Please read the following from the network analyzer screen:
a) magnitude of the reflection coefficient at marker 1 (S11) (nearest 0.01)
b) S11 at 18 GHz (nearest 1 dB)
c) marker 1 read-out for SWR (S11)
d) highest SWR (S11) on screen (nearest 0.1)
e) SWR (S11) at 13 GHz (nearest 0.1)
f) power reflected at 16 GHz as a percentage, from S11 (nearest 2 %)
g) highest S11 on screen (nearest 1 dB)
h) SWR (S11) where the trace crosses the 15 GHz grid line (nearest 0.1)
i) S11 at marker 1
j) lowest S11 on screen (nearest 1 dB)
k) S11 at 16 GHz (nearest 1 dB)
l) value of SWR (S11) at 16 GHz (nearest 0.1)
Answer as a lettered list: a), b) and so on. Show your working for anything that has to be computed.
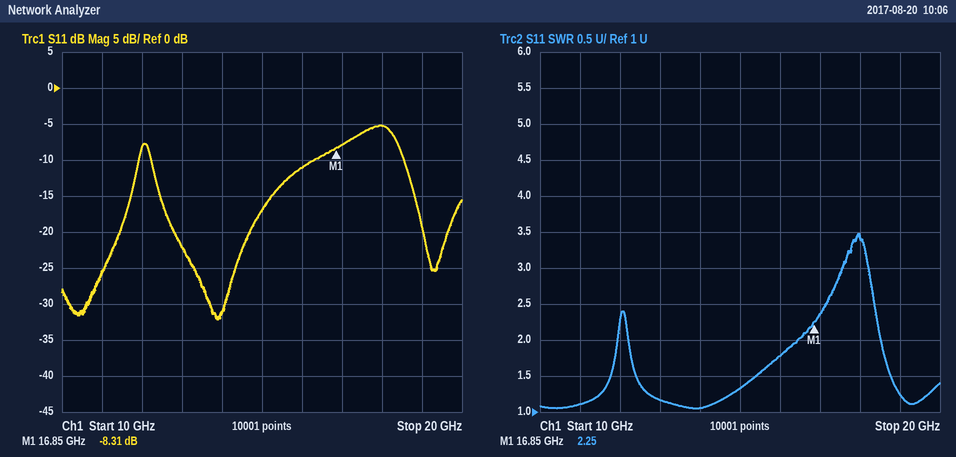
a) 10^(-8.31/20) ≈ 0.38
b) -5 dB
c) 2.25
d) 3.5
e) 1.2
f) 10^(-11/10) ≈ 8 %
g) -5 dB
h) 1.3
i) -8.31 dB
j) -32 dB
k) -11 dB
l) 1.8
